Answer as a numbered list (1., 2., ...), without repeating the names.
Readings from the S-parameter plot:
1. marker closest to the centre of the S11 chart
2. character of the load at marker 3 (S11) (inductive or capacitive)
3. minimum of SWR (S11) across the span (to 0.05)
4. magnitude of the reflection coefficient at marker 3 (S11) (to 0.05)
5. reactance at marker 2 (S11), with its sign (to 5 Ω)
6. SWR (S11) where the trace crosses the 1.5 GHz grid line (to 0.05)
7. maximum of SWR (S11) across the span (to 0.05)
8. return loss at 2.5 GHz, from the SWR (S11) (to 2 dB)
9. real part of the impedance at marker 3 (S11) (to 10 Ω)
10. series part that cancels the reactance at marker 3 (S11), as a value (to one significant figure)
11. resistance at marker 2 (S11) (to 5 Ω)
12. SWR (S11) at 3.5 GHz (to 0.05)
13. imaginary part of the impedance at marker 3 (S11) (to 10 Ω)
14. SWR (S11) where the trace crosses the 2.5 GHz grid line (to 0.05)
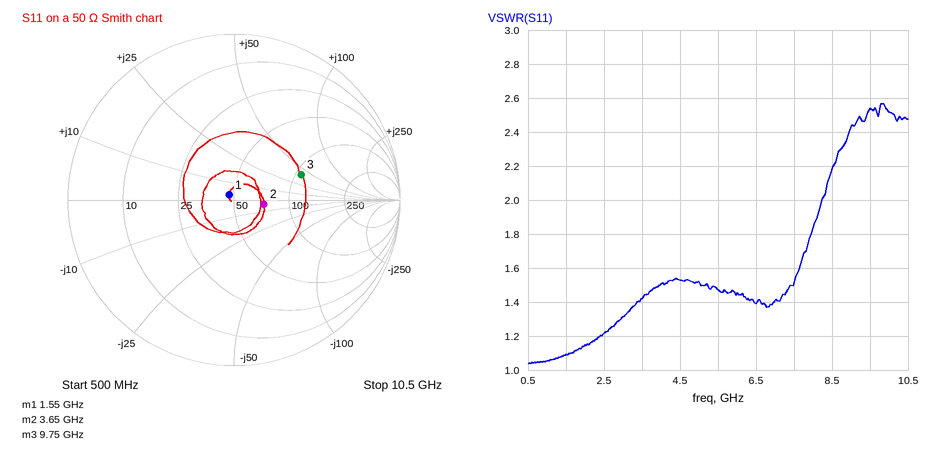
1. marker 1
2. inductive
3. 1.05
4. 0.45
5. -5 Ω
6. 1.10
7. 2.55
8. 20 dB
9. 110 Ω
10. 400 fF
11. 70 Ω
12. 1.40
13. +40 Ω
14. 1.20
